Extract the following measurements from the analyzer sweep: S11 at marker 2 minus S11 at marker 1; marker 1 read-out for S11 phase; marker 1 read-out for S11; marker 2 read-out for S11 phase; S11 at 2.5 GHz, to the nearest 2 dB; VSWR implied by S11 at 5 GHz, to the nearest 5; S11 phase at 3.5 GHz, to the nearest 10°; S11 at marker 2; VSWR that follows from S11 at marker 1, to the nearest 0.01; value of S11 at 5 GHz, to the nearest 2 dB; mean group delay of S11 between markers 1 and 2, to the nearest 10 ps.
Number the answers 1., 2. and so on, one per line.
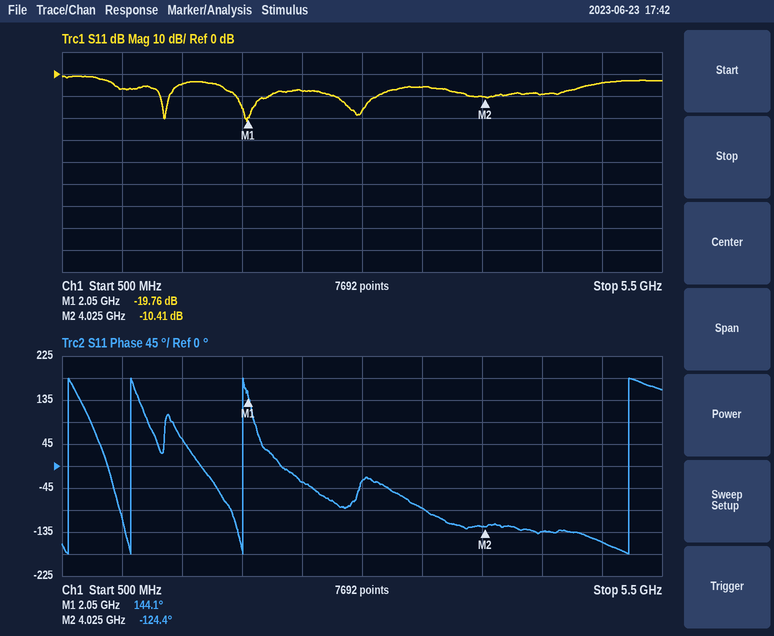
1. 9.35 dB
2. 144.1°
3. -19.76 dB
4. -124.4°
5. -8 dB
6. 5
7. -90°
8. -10.41 dB
9. 1.23
10. -4 dB
11. 380 ps
